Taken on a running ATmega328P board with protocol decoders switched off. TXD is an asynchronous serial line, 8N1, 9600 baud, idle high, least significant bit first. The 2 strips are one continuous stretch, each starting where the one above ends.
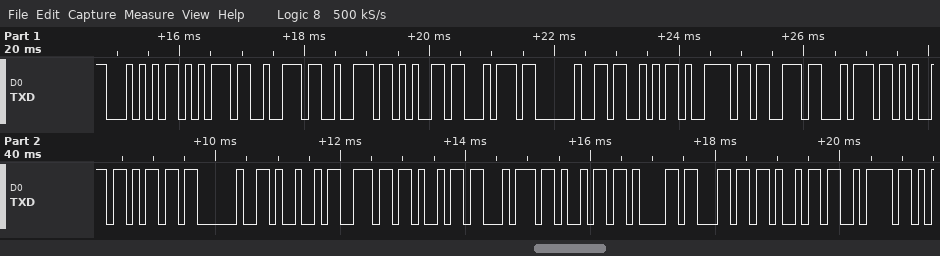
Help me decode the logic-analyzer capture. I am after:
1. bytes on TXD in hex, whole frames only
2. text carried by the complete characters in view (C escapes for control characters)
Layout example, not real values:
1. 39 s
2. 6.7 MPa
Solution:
1. 54 75 72 72 65 74 20 53 79 73 74 65 6D 20 49 6E 69 74 69 61 6C 69 7A
2. "Turret System Initializ"
